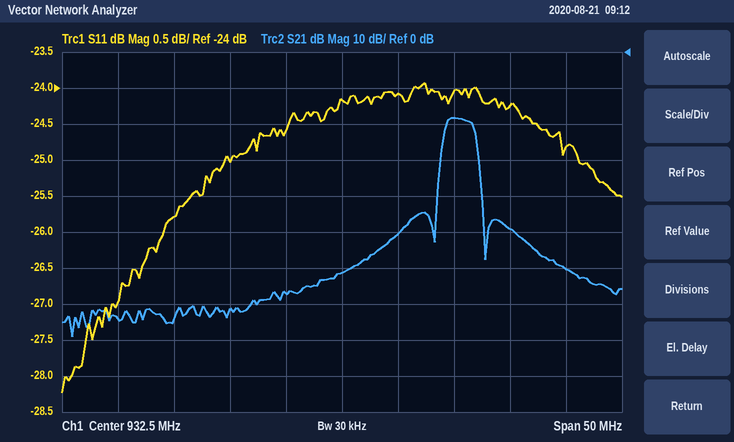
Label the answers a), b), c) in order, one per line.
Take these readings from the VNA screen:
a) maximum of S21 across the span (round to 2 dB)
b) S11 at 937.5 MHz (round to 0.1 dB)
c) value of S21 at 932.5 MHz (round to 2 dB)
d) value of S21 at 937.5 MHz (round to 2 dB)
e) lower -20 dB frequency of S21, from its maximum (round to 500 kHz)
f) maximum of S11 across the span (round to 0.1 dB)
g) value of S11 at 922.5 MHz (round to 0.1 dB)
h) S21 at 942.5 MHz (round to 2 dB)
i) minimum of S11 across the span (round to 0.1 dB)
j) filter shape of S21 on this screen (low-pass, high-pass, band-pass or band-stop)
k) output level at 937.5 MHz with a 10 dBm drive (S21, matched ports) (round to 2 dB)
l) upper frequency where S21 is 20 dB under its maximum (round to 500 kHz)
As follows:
a) -18 dB
b) -24.1 dB
c) -62 dB
d) -50 dB
e) 941.0 MHz
f) -23.9 dB
g) -25.0 dB
h) -18 dB
i) -28.2 dB
j) band-pass
k) -40 dBm
l) 945.0 MHz
